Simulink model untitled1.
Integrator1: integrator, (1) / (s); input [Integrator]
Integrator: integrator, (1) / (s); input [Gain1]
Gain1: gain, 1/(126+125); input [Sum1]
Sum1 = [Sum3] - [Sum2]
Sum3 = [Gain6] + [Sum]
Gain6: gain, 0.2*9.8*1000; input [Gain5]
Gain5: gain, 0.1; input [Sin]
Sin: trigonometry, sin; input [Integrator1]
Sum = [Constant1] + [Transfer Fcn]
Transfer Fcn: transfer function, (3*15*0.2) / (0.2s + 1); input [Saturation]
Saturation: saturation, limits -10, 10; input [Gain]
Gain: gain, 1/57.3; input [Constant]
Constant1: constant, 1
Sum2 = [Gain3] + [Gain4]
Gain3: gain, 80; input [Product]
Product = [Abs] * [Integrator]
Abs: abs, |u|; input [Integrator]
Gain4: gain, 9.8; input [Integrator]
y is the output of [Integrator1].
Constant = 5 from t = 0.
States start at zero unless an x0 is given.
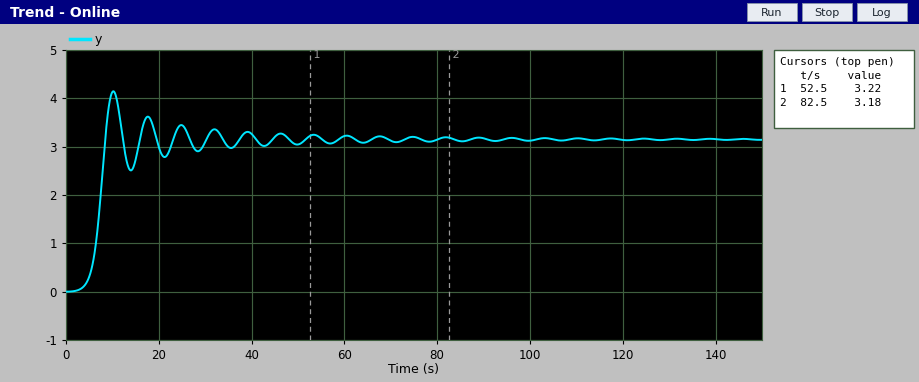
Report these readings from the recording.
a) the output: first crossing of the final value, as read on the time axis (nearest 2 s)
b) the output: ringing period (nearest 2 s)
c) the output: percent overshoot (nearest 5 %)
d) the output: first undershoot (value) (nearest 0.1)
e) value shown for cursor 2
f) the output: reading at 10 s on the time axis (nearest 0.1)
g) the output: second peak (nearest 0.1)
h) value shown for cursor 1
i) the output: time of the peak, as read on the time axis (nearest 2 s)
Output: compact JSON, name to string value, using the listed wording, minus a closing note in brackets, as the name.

{"the output: first crossing of the final value, as read on the time axis": "8 s", "the output: ringing period": "8 s", "the output: percent overshoot": "30 %", "the output: first undershoot (value)": "2.5", "value shown for cursor 2": "3.18", "the output: reading at 10 s on the time axis": "4.1", "the output: second peak": "3.6", "value shown for cursor 1": "3.22", "the output: time of the peak, as read on the time axis": "10 s"}
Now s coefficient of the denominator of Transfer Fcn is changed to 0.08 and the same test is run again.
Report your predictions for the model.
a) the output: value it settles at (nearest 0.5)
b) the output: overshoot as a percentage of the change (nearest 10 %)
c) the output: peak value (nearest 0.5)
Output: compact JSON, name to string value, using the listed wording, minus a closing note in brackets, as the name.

{"the output: value it settles at": "3.0", "the output: overshoot as a percentage of the change": "30 %", "the output: peak value": "4.0"}
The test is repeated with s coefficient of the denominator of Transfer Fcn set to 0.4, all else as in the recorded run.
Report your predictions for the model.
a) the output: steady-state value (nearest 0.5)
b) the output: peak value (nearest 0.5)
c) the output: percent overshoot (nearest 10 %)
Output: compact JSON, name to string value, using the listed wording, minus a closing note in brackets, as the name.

{"the output: steady-state value": "3.0", "the output: peak value": "4.0", "the output: percent overshoot": "30 %"}
